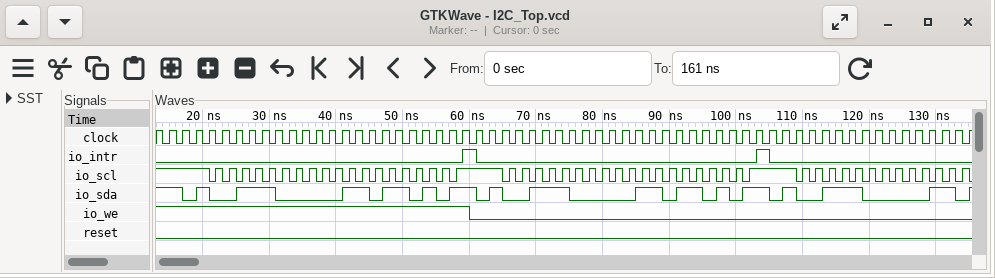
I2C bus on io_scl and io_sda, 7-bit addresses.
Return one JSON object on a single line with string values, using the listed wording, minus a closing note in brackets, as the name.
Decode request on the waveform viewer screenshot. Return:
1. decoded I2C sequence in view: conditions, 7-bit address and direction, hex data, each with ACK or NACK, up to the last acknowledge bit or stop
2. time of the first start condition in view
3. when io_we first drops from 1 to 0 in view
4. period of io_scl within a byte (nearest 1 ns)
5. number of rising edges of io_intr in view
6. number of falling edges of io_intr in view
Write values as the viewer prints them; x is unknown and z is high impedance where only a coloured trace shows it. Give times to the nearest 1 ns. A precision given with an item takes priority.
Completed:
{"decoded I2C sequence in view: conditions, 7-bit address and direction, hex data, each with ACK or NACK, up to the last acknowledge bit or stop": "start, address 1C write ACK, 6D ACK, repeated start, address 1C write ACK, 6D ACK, repeated start, address 1C write ACK", "time of the first start condition in view": "17 ns", "when io_we first drops from 1 to 0 in view": "60 ns", "period of io_scl within a byte": "2 ns", "number of rising edges of io_intr in view": "2", "number of falling edges of io_intr in view": "2"}
